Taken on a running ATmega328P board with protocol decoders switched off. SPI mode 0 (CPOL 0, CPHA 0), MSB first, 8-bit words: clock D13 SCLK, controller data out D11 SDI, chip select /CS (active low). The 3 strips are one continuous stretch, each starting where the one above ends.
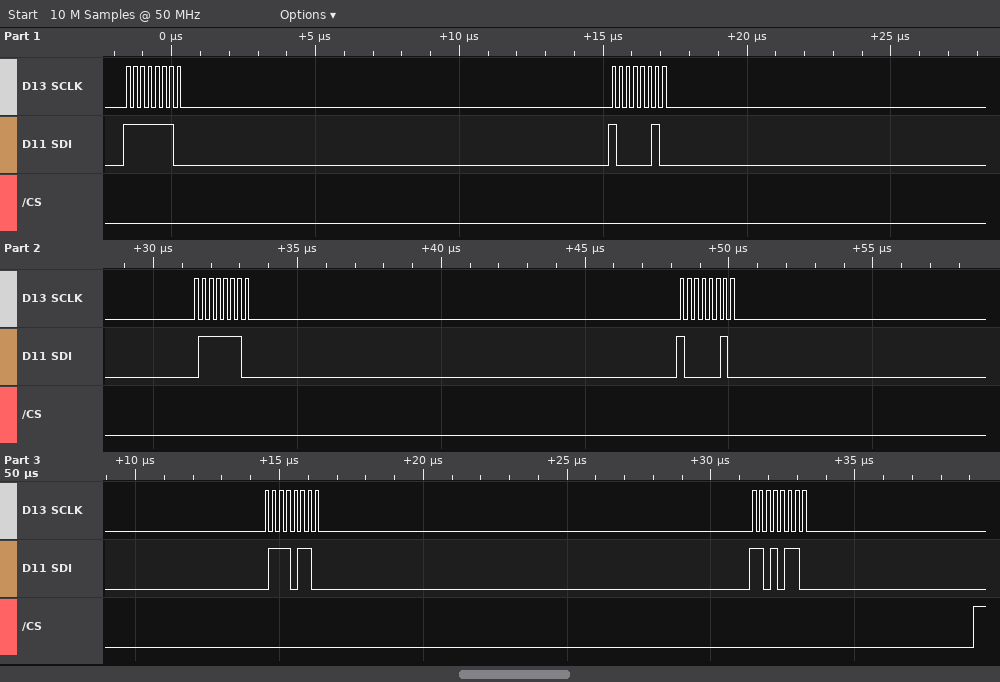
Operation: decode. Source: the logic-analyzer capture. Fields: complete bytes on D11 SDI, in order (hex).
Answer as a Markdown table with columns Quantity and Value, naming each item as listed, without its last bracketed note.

| Quantity | Value |
|---|---|
| complete bytes on D11 SDI, in order | FE 82 7E 82 76 D6 |
